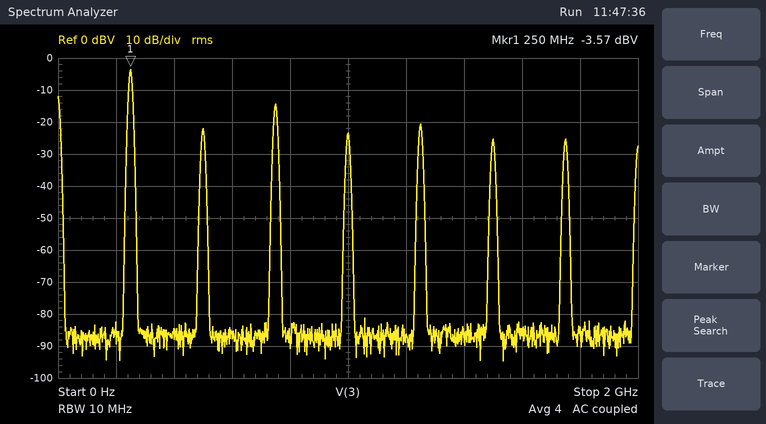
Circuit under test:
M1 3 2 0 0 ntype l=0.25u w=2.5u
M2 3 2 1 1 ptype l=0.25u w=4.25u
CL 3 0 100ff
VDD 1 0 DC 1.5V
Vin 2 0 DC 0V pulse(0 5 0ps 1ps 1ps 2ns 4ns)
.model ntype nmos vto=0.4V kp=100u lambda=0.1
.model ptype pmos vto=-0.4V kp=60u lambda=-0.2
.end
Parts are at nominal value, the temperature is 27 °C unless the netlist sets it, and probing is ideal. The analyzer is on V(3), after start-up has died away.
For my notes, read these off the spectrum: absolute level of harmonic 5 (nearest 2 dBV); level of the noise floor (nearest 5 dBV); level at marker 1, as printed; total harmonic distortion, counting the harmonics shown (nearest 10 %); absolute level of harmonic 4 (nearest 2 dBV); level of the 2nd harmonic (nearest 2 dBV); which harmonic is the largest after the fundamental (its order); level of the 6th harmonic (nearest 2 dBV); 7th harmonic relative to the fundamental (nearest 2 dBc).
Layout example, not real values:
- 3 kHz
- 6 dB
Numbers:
- -20 dBV
- -85 dBV
- -3.57 dBV
- 40 %
- -24 dBV
- -22 dBV
- 3
- -26 dBV
- -22 dBc
